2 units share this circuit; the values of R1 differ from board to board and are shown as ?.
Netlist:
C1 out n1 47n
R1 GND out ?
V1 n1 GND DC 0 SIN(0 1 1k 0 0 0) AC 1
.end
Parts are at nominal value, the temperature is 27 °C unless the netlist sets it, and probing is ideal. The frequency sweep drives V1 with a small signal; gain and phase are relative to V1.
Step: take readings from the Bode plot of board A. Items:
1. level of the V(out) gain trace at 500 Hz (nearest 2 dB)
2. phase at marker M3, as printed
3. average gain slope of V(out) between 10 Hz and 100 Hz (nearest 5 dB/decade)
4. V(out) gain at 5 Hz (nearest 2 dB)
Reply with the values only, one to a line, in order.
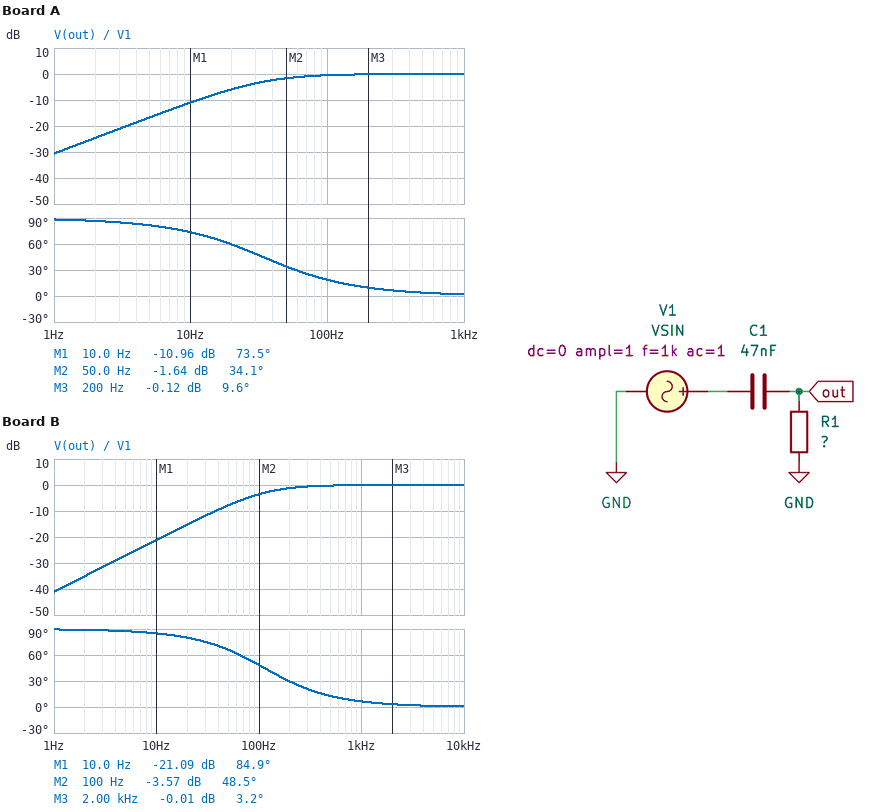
0 dB
9.6 deg
10 dB/decade
-16 dB
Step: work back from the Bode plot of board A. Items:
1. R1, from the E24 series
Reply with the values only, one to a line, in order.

100 kΩ
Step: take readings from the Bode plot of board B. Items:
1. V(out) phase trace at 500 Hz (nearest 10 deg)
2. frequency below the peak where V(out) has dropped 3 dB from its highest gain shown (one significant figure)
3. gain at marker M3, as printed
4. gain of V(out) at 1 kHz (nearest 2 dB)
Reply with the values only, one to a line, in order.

10 deg
100 Hz
-0.01 dB
0 dB
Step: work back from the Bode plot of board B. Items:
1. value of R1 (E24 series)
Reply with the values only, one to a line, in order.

30 kΩ
